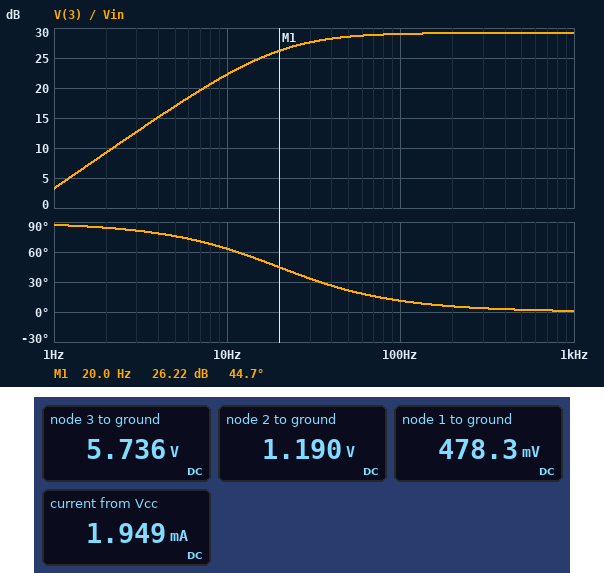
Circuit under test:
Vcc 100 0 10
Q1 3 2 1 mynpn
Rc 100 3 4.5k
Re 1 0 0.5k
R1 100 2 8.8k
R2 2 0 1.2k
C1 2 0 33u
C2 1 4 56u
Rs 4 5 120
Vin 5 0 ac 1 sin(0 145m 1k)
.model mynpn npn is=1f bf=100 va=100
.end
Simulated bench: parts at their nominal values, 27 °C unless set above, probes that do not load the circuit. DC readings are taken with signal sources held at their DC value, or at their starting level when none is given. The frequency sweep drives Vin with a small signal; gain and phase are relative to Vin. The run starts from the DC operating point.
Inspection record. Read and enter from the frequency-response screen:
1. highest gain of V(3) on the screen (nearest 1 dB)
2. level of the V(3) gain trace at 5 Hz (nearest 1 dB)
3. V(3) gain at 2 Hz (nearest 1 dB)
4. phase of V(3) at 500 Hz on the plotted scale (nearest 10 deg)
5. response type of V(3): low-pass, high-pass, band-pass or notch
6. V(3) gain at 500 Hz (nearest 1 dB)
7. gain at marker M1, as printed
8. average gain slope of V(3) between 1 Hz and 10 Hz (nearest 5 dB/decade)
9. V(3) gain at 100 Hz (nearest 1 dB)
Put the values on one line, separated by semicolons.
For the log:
29 dB; 17 dB; 9 dB; 0 deg; high-pass; 29 dB; 26.22 dB; 20 dB/decade; 29 dB
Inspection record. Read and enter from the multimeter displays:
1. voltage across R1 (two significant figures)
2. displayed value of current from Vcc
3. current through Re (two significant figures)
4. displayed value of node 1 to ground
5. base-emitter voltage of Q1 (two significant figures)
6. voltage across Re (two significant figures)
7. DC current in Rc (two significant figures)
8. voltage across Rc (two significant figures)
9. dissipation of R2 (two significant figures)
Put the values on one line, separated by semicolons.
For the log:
8.8 V; 1.949 mA; 960 µA; 478.3 mV; 710 mV; 480 mV; 950 µA; 4.3 V; 1.2 mW
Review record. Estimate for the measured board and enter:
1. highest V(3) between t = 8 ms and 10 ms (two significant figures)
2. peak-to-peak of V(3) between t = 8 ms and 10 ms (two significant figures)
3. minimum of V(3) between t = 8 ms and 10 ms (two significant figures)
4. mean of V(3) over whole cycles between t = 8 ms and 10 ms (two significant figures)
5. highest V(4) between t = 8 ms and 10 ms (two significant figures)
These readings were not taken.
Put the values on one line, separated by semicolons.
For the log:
9.2 V; 7.8 V; 1.4 V; 5.6 V; 41 mV
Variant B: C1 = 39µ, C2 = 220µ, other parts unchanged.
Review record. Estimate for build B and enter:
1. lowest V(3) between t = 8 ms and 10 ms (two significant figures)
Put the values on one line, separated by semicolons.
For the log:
1.3 V
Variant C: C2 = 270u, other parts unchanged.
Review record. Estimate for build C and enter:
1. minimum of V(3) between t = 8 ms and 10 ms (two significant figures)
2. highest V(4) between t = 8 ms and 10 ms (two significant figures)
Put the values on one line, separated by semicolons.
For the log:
1.3 V; 42 mV
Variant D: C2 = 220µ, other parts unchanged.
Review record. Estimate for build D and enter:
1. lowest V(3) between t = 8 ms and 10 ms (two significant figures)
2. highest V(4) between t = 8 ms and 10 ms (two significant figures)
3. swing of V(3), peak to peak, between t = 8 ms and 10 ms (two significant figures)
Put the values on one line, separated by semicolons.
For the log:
1.3 V; 42 mV; 7.9 V
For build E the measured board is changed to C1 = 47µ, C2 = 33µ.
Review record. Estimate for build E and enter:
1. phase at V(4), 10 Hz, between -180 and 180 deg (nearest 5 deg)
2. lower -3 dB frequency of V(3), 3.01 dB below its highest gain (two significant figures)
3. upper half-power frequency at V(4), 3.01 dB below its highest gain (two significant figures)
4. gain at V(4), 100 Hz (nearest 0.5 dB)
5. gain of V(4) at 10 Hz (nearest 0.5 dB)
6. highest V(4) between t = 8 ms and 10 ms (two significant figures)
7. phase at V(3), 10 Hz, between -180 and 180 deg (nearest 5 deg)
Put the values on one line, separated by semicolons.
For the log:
-15 deg; 33 Hz; 34 Hz; -9.0 dB; -0.5 dB; 40 mV; 75 deg
